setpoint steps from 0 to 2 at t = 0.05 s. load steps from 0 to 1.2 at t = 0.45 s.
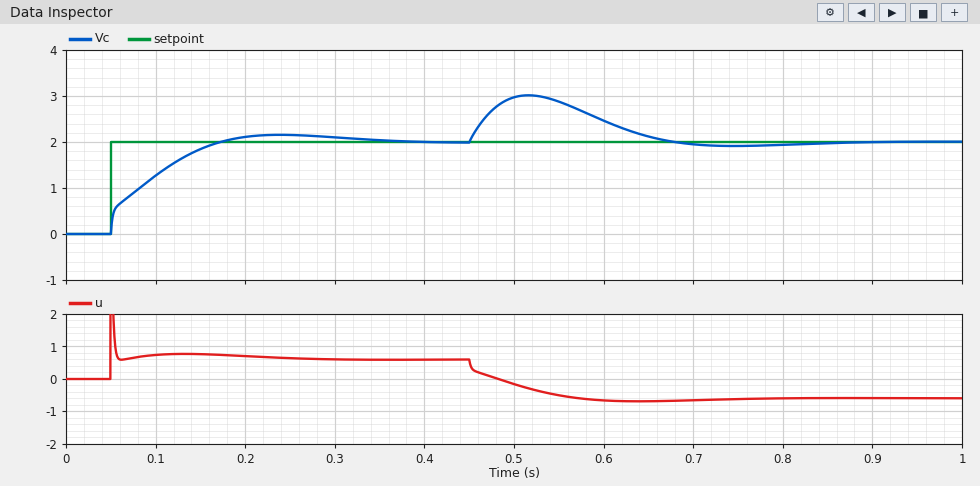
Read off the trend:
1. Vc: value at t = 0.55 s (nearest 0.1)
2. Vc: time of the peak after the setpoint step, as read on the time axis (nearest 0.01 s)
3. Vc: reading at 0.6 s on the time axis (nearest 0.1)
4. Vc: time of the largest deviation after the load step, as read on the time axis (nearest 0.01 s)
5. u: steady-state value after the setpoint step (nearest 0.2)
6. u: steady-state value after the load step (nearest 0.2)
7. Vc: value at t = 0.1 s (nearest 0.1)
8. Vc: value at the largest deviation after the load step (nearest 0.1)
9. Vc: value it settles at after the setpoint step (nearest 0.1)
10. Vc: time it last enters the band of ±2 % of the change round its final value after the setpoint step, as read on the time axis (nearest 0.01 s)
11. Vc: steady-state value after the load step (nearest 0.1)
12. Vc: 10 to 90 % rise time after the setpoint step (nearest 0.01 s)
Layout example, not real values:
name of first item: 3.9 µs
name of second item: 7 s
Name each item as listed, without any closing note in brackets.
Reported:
Vc: value at t = 0.55 s: 2.9
Vc: time of the peak after the setpoint step, as read on the time axis: 0.24 s
Vc: reading at 0.6 s on the time axis: 2.5
Vc: time of the largest deviation after the load step, as read on the time axis: 0.52 s
u: steady-state value after the setpoint step: 0.6
u: steady-state value after the load step: -0.6
Vc: value at t = 0.1 s: 1.3
Vc: value at the largest deviation after the load step: 3.0
Vc: value it settles at after the setpoint step: 2.0
Vc: time it last enters the band of ±2 % of the change round its final value after the setpoint step, as read on the time axis: 0.35 s
Vc: steady-state value after the load step: 2.0
Vc: 10 to 90 % rise time after the setpoint step: 0.09 s
